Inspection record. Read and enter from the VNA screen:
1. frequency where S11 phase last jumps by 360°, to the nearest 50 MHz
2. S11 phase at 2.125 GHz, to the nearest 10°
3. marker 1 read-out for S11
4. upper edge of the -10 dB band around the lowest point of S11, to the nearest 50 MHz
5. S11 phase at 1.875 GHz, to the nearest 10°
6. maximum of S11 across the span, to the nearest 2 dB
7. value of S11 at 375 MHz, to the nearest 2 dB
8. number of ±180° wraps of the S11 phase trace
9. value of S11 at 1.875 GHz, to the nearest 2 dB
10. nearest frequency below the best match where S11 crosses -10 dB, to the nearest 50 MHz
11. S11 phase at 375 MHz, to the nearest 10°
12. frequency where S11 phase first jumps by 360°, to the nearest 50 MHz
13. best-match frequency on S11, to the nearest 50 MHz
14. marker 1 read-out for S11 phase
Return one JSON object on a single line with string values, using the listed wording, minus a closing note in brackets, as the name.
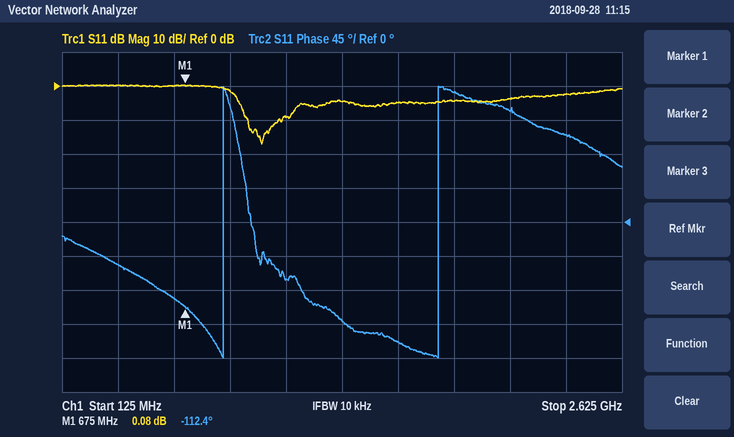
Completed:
{"frequency where S11 phase last jumps by 360°, to the nearest 50 MHz": "1.80 GHz", "S11 phase at 2.125 GHz, to the nearest 10°": "150°", "marker 1 read-out for S11": "0.08 dB", "upper edge of the -10 dB band around the lowest point of S11, to the nearest 50 MHz": "1.10 GHz", "S11 phase at 1.875 GHz, to the nearest 10°": "170°", "maximum of S11 across the span, to the nearest 2 dB": "0 dB", "value of S11 at 375 MHz, to the nearest 2 dB": "0 dB", "number of ±180° wraps of the S11 phase trace": "2", "value of S11 at 1.875 GHz, to the nearest 2 dB": "-4 dB", "nearest frequency below the best match where S11 crosses -10 dB, to the nearest 50 MHz": "950 MHz", "S11 phase at 375 MHz, to the nearest 10°": "-60°", "frequency where S11 phase first jumps by 360°, to the nearest 50 MHz": "850 MHz", "best-match frequency on S11, to the nearest 50 MHz": "1.00 GHz", "marker 1 read-out for S11 phase": "-112.4°"}
